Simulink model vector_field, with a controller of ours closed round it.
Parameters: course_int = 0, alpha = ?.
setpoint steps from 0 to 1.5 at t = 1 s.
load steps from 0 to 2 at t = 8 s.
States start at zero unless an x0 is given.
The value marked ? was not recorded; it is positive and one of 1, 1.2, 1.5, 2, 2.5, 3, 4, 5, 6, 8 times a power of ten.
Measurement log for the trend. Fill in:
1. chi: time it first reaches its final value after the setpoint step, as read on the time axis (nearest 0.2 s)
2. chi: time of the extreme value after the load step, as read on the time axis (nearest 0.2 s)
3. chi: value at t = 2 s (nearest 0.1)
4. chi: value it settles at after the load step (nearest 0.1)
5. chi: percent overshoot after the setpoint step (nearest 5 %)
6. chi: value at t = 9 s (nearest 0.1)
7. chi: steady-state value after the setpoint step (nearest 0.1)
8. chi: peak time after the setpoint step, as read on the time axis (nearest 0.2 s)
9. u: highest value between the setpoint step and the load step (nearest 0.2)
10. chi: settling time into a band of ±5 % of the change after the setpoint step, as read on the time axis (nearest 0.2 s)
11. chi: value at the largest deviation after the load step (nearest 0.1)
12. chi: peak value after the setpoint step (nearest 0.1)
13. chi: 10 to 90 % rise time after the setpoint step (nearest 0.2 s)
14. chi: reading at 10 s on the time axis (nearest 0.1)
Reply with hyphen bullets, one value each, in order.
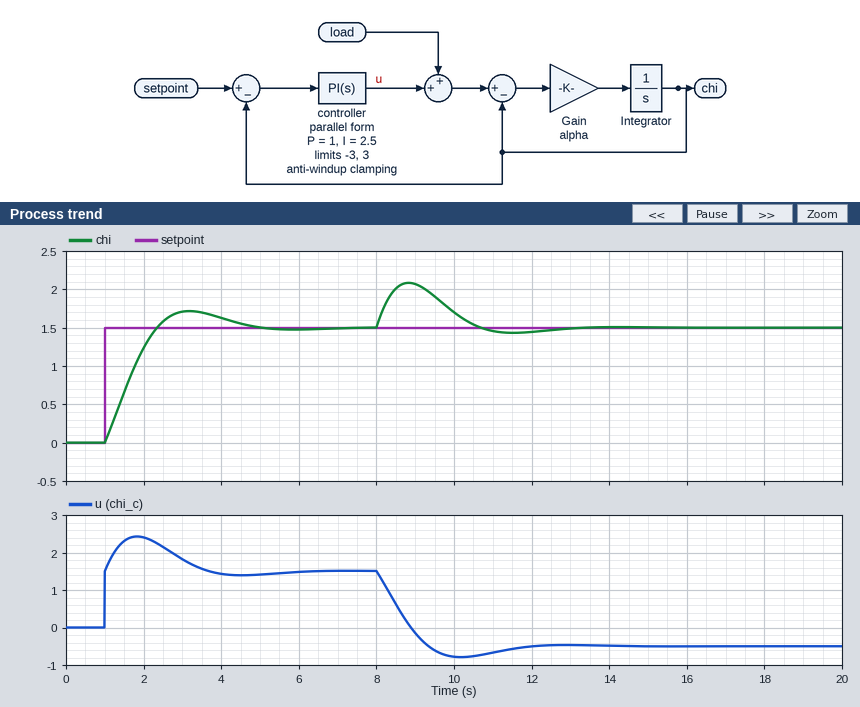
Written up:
- 2.4 s
- 8.8 s
- 1.2
- 1.5
- 15 %
- 2.1
- 1.5
- 3.2 s
- 2.4
- 4.4 s
- 2.1
- 1.7
- 1.0 s
- 1.7
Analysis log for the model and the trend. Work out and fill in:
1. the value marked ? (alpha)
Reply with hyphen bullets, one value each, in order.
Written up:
- 0.8
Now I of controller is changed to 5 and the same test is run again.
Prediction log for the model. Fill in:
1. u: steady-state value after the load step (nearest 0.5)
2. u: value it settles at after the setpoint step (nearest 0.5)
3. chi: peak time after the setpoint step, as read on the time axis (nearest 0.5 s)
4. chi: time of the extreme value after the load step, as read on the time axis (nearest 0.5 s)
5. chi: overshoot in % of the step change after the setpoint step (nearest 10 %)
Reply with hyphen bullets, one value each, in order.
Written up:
- -0.5
- 1.5
- 2.5 s
- 8.5 s
- 20 %
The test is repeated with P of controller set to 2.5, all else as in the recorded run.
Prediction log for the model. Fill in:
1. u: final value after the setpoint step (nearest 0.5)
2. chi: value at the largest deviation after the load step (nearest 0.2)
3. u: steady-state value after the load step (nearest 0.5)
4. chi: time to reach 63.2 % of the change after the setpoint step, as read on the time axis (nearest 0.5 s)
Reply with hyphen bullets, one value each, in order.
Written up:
- 1.5
- 2.0
- -0.5
- 1.5 s
